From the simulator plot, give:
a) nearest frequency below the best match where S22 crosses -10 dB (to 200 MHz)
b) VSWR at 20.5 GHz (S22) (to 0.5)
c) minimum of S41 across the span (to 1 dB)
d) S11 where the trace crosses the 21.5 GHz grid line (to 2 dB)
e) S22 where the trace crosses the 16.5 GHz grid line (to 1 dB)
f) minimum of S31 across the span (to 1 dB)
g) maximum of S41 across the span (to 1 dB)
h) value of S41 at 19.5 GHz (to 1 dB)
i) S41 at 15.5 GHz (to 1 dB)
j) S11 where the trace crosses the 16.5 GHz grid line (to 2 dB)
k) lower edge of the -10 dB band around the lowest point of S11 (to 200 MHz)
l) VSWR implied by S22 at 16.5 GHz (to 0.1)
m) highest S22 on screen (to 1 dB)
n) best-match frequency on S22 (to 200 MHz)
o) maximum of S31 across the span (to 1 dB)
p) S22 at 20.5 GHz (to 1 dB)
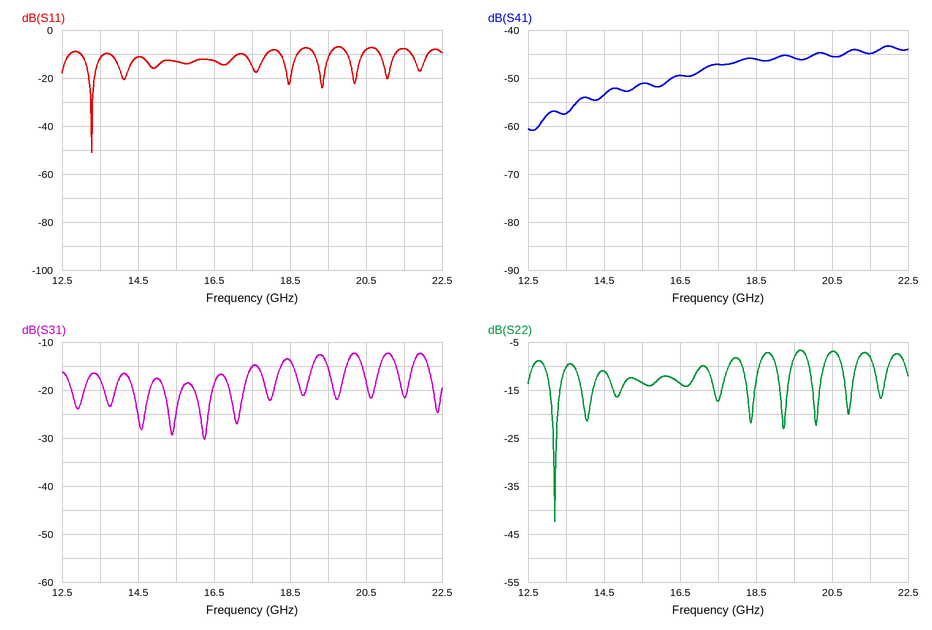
13.0 GHz
2.5
-61 dB
-8 dB
-14 dB
-30 dB
-43 dB
-46 dB
-51 dB
-12 dB
13.0 GHz
1.5
-7 dB
13.2 GHz
-12 dB
-7 dB
